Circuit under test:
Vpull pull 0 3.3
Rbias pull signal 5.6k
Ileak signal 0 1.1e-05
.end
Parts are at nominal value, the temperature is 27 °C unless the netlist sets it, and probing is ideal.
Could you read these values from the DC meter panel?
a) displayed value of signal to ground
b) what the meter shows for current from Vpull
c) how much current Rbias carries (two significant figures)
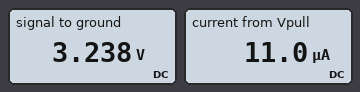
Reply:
3.238 V
11.0 µA
11 µA
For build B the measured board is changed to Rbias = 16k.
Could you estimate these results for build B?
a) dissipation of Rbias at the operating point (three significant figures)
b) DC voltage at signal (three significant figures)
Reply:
1.94 µW
3.12 V
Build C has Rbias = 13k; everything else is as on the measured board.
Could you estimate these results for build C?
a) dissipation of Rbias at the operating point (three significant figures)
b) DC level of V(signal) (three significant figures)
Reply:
1.57 µW
3.16 V
